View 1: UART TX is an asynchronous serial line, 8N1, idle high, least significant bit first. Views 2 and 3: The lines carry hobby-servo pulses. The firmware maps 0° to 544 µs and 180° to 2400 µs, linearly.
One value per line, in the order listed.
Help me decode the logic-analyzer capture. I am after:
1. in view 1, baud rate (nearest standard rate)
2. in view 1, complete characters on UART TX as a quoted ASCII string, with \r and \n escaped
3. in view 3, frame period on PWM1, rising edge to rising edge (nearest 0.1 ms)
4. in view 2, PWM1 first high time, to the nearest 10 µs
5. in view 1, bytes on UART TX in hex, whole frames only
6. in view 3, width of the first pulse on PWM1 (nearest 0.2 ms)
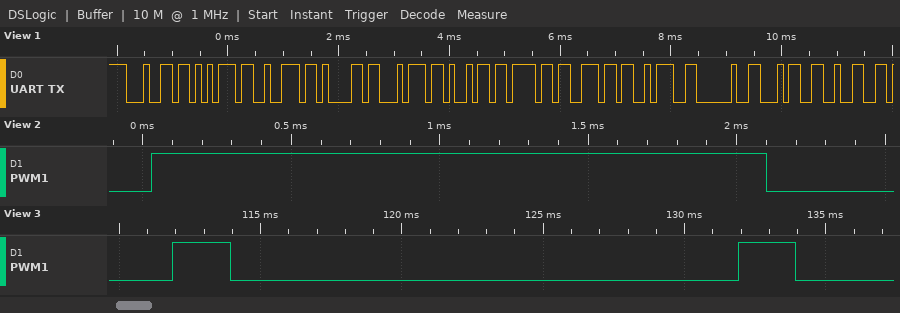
9600 baud
"duration: 42"
20.0 ms
2070 µs
64 75 72 61 74 69 6F 6E 3A 20 34 32
2.0 ms
